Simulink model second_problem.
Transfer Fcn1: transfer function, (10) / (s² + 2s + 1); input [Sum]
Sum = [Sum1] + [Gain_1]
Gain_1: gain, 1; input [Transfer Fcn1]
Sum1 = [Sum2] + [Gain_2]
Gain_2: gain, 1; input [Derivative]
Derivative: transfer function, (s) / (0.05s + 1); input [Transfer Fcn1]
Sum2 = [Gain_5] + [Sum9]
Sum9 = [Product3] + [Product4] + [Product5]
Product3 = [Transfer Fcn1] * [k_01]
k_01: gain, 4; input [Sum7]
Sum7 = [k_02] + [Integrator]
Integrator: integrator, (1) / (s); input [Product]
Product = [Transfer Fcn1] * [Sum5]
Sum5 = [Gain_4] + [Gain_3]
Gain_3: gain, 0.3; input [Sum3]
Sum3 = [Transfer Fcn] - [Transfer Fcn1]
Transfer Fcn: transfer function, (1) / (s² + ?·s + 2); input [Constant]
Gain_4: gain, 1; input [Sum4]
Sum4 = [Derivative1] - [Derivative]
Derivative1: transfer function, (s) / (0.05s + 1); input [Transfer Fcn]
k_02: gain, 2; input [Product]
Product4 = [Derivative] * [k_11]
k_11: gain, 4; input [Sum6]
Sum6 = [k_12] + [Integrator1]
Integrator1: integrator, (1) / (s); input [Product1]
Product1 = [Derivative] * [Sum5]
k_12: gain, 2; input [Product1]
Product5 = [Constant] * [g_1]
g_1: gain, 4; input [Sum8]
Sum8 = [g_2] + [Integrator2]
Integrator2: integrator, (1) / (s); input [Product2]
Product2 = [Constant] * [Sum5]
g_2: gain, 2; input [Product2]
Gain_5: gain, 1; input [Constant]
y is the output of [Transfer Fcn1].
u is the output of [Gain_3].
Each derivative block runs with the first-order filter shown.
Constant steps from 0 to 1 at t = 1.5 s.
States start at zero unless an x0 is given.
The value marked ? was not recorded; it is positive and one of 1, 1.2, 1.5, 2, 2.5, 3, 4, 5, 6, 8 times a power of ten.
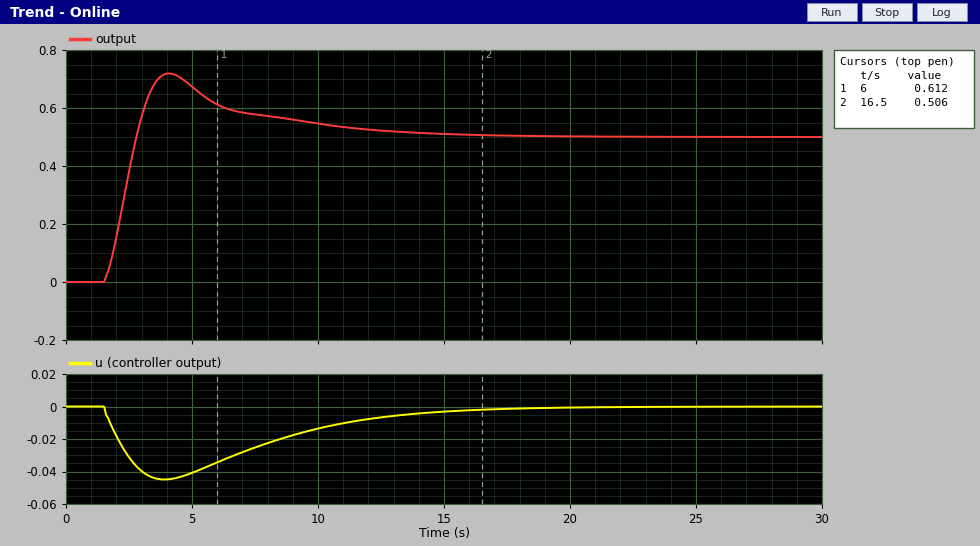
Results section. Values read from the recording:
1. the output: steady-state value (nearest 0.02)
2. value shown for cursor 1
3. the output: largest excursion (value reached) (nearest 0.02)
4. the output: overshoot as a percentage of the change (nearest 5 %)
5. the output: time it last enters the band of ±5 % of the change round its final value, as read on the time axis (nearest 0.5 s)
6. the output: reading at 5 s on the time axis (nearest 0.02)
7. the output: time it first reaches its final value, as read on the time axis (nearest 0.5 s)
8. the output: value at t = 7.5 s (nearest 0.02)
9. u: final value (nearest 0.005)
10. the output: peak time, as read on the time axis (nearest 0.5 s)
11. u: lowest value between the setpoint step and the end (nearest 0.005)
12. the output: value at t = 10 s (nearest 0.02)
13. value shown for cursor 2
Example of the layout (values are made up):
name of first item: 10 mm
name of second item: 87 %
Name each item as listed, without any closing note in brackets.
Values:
the output: steady-state value: 0.50
value shown for cursor 1: 0.612
the output: largest excursion (value reached): 0.72
the output: overshoot as a percentage of the change: 45 %
the output: time it last enters the band of ±5 % of the change round its final value, as read on the time axis: 12.0 s
the output: reading at 5 s on the time axis: 0.68
the output: time it first reaches its final value, as read on the time axis: 3.0 s
the output: value at t = 7.5 s: 0.58
u: final value: 0.000
the output: peak time, as read on the time axis: 4.0 s
u: lowest value between the setpoint step and the end: -0.045
the output: value at t = 10 s: 0.54
value shown for cursor 2: 0.506
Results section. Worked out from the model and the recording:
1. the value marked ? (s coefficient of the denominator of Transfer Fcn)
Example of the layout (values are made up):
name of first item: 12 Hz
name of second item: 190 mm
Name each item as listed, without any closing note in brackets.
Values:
the value marked ?: 1.5
